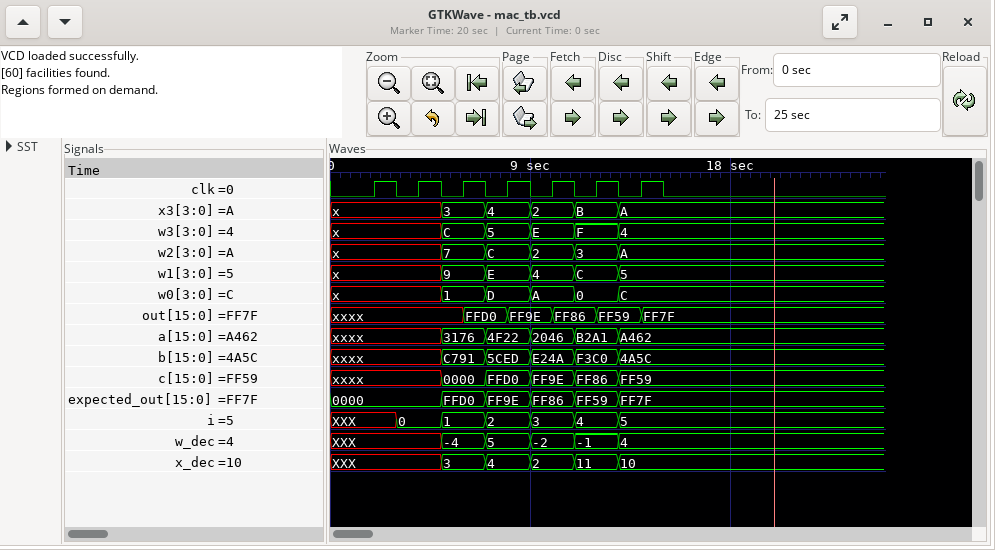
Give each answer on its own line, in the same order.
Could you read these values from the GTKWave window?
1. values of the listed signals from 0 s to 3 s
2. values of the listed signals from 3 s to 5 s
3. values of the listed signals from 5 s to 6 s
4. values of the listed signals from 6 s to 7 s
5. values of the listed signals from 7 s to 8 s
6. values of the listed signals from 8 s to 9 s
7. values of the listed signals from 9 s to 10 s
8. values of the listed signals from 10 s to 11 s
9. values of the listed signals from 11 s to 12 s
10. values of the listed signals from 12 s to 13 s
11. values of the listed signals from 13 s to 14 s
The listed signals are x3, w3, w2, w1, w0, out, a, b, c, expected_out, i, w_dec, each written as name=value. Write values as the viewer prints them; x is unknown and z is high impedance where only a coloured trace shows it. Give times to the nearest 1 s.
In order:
x3=x, w3=x, w2=x, w1=x, w0=x, out=xxxx, a=xxxx, b=xxxx, c=xxxx, expected_out=0000, i=XXX, w_dec=XXX
x3=x, w3=x, w2=x, w1=x, w0=x, out=xxxx, a=xxxx, b=xxxx, c=xxxx, expected_out=0000, i=0, w_dec=XXX
x3=3, w3=C, w2=7, w1=9, w0=1, out=xxxx, a=3176, b=C791, c=0000, expected_out=FFD0, i=1, w_dec=-4
x3=3, w3=C, w2=7, w1=9, w0=1, out=FFD0, a=3176, b=C791, c=0000, expected_out=FFD0, i=1, w_dec=-4
x3=4, w3=5, w2=C, w1=E, w0=D, out=FFD0, a=4F22, b=5CED, c=FFD0, expected_out=FF9E, i=2, w_dec=5
x3=4, w3=5, w2=C, w1=E, w0=D, out=FF9E, a=4F22, b=5CED, c=FFD0, expected_out=FF9E, i=2, w_dec=5
x3=2, w3=E, w2=2, w1=4, w0=A, out=FF9E, a=2046, b=E24A, c=FF9E, expected_out=FF86, i=3, w_dec=-2
x3=2, w3=E, w2=2, w1=4, w0=A, out=FF86, a=2046, b=E24A, c=FF9E, expected_out=FF86, i=3, w_dec=-2
x3=B, w3=F, w2=3, w1=C, w0=0, out=FF86, a=B2A1, b=F3C0, c=FF86, expected_out=FF59, i=4, w_dec=-1
x3=B, w3=F, w2=3, w1=C, w0=0, out=FF59, a=B2A1, b=F3C0, c=FF86, expected_out=FF59, i=4, w_dec=-1
x3=A, w3=4, w2=A, w1=5, w0=C, out=FF59, a=A462, b=4A5C, c=FF59, expected_out=FF7F, i=5, w_dec=4
